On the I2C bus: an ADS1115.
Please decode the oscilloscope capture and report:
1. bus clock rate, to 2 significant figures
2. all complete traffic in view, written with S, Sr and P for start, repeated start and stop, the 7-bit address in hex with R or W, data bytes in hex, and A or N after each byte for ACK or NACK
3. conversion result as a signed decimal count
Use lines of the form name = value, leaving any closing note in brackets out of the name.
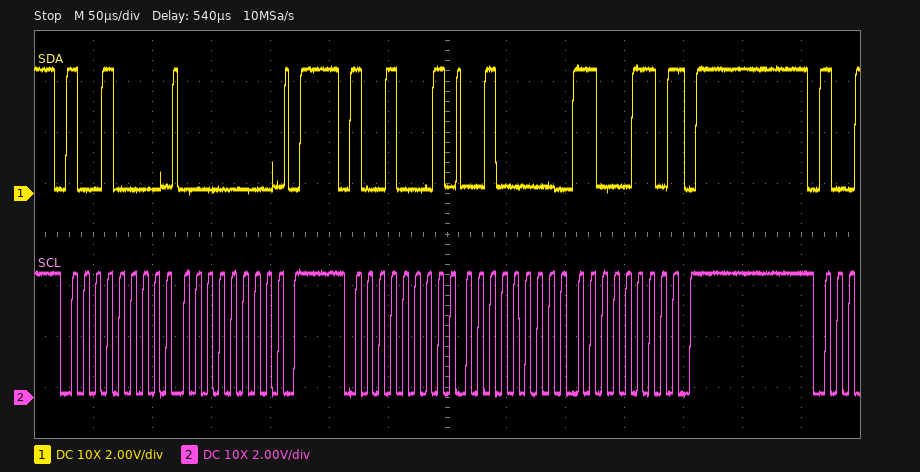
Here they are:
bus clock rate, to 2 significant figures = 100 kHz
all complete traffic in view, written with S, Sr and P for start, repeated start and stop, the 7-bit address in hex with R or W, data bytes in hex, and A or N after each byte for ACK or NACK = S 48W A 00 A P S 48R A 20 A C6 N P
conversion result as a signed decimal count = 8390
